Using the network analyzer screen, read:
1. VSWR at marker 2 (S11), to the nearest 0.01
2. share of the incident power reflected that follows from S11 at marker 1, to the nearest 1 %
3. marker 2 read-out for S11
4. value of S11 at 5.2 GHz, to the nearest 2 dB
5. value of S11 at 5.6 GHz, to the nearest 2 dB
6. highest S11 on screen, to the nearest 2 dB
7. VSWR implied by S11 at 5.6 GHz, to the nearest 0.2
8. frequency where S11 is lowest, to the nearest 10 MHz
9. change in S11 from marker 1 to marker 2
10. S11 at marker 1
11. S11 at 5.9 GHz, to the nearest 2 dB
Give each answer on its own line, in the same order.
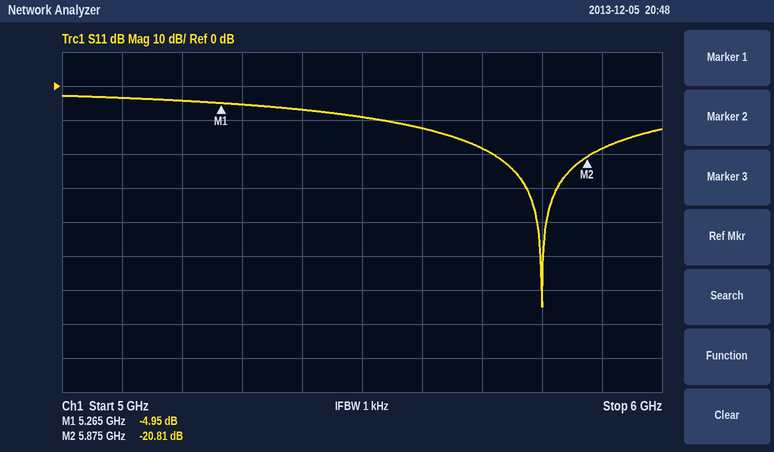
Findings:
1.20
32 %
-20.81 dB
-4 dB
-12 dB
-2 dB
1.6
5.80 GHz
-15.86 dB
-4.95 dB
-18 dB
